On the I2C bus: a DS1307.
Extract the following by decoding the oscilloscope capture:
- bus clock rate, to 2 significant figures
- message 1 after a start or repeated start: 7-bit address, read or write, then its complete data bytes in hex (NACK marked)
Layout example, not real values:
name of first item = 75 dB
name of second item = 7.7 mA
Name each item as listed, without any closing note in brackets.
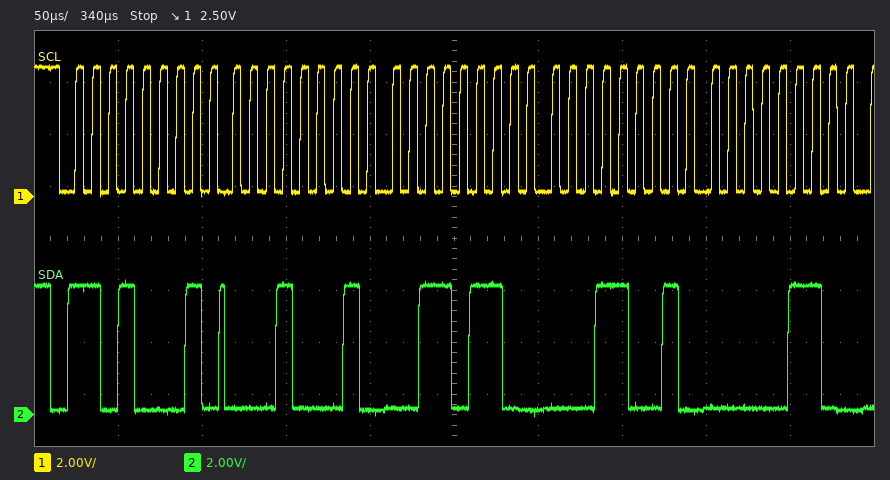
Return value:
bus clock rate, to 2 significant figures = 100 kHz
message 1 after a start or repeated start: 7-bit address, read or write, then its complete data bytes in hex = 0x68 read: 11 36 19 06
